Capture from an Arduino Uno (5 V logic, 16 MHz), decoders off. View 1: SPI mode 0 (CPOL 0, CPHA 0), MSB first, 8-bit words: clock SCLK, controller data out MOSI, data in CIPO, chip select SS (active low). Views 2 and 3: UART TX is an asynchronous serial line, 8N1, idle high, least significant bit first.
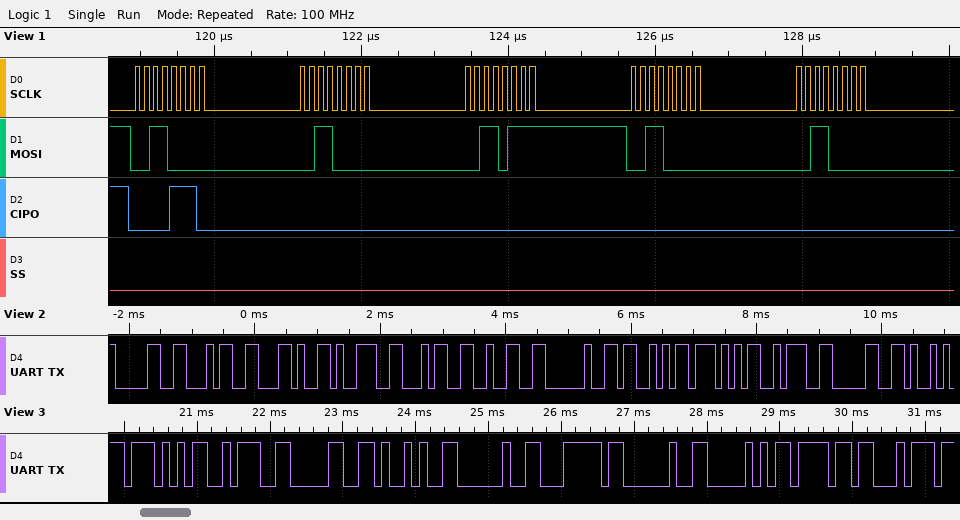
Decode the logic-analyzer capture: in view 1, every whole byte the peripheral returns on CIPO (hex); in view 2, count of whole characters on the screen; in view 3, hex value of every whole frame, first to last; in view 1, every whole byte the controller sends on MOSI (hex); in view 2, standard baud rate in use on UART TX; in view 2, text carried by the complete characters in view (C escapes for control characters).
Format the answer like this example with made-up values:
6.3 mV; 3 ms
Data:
0E 00 00 00 00; 11; 0x57 0x3A 0x30 0x29 0x20 0x7C 0x20 0x50 0x6F 0x74; 30 30 37 30 30; 9600 baud; "04,942 SW:0"
